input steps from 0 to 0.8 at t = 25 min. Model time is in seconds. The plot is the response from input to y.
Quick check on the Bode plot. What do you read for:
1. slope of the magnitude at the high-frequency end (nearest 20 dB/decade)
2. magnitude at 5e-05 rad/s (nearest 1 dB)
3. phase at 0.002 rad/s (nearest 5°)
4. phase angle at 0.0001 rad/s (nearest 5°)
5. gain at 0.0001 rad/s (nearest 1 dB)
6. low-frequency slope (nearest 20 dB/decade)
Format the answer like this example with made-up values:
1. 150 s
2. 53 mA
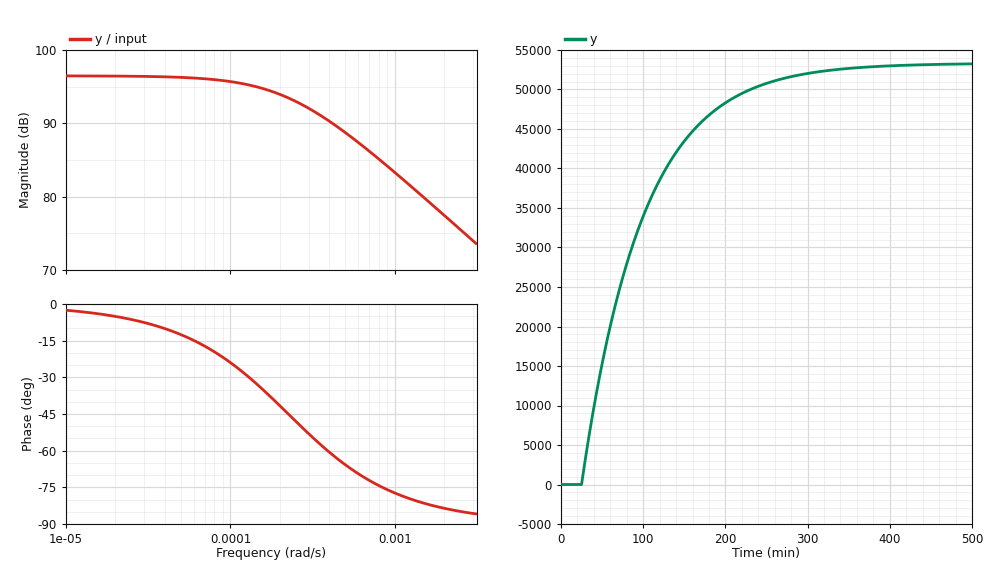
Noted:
1. -20 dB/decade
2. 96 dB
3. -85°
4. -25°
5. 96 dB
6. 0 dB/decade
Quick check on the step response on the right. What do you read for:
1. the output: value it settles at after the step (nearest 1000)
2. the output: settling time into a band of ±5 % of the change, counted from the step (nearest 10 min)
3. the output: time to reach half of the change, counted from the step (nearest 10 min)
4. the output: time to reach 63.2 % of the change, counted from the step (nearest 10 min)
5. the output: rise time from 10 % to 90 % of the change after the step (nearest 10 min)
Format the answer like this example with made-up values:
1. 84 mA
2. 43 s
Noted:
1. 53000
2. 220 min
3. 50 min
4. 70 min
5. 160 min
